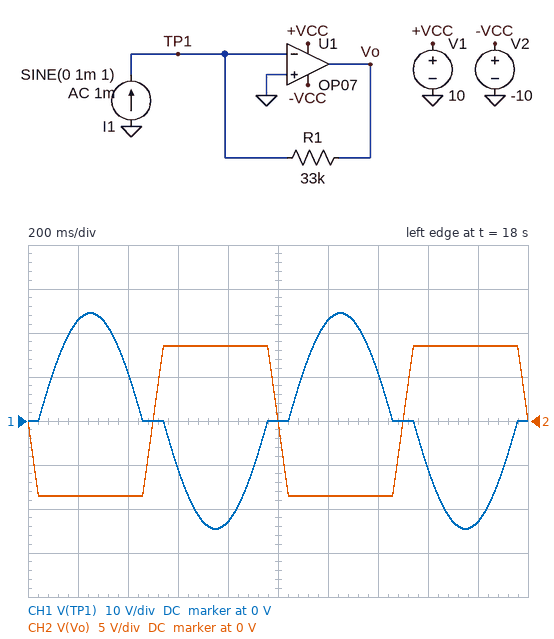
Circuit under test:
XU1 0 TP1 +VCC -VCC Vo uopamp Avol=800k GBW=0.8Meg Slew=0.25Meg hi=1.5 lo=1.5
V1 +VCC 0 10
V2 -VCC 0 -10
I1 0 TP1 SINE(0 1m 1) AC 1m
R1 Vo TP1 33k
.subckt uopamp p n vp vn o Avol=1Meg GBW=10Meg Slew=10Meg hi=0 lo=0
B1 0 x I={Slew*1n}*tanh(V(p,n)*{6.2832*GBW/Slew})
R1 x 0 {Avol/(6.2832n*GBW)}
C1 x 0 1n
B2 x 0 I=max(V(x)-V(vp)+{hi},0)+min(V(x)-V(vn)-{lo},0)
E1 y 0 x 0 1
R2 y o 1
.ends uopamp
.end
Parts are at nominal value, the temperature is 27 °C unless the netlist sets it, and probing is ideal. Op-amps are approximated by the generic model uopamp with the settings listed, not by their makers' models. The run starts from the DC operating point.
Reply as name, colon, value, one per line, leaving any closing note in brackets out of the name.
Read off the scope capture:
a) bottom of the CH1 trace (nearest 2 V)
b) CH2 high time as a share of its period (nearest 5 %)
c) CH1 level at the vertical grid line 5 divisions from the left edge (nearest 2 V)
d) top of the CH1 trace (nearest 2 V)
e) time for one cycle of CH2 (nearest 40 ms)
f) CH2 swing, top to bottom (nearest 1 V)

bottom of the CH1 trace: -24 V
CH2 high time as a share of its period: 50 %
CH1 level at the vertical grid line 5 divisions from the left edge: 0 V
top of the CH1 trace: 24 V
time for one cycle of CH2: 1.00 s
CH2 swing, top to bottom: 17 V
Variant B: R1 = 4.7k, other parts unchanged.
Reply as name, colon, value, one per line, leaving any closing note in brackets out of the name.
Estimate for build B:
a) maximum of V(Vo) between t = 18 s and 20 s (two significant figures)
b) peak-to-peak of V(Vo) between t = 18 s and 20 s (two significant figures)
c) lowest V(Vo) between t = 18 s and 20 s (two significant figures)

maximum of V(Vo) between t = 18 s and 20 s: 4.7 V
peak-to-peak of V(Vo) between t = 18 s and 20 s: 9.4 V
lowest V(Vo) between t = 18 s and 20 s: -4.7 V
